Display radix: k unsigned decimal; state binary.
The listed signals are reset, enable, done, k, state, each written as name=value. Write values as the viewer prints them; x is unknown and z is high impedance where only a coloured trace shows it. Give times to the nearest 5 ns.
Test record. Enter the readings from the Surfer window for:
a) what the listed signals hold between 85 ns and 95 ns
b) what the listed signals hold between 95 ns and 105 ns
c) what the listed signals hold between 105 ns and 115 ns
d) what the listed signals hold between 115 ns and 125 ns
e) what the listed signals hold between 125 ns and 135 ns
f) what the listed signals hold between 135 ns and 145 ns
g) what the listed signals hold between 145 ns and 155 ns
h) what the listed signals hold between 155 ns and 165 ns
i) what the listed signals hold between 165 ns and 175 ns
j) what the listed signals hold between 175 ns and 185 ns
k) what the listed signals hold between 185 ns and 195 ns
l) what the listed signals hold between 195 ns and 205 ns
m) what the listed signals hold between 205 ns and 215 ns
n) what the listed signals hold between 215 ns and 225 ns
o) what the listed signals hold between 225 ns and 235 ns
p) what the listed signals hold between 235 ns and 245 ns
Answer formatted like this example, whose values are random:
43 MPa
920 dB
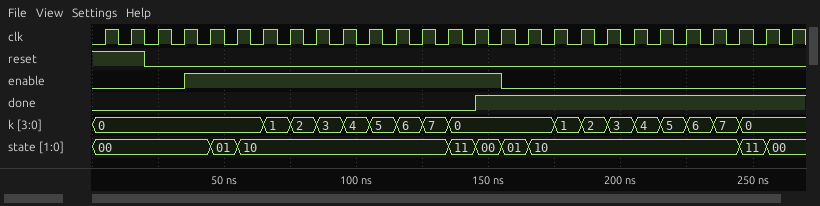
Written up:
reset=0, enable=1, done=0, k=3, state=10
reset=0, enable=1, done=0, k=4, state=10
reset=0, enable=1, done=0, k=5, state=10
reset=0, enable=1, done=0, k=6, state=10
reset=0, enable=1, done=0, k=7, state=10
reset=0, enable=1, done=0, k=0, state=11
reset=0, enable=1, done=1, k=0, state=00
reset=0, enable=0, done=1, k=0, state=01
reset=0, enable=0, done=1, k=0, state=10
reset=0, enable=0, done=1, k=1, state=10
reset=0, enable=0, done=1, k=2, state=10
reset=0, enable=0, done=1, k=3, state=10
reset=0, enable=0, done=1, k=4, state=10
reset=0, enable=0, done=1, k=5, state=10
reset=0, enable=0, done=1, k=6, state=10
reset=0, enable=0, done=1, k=7, state=10
